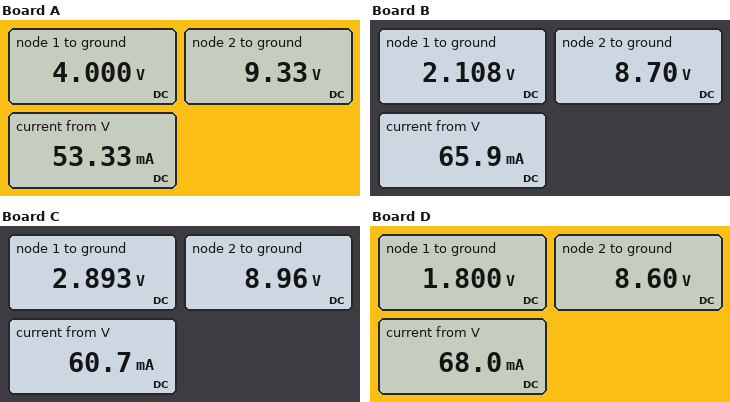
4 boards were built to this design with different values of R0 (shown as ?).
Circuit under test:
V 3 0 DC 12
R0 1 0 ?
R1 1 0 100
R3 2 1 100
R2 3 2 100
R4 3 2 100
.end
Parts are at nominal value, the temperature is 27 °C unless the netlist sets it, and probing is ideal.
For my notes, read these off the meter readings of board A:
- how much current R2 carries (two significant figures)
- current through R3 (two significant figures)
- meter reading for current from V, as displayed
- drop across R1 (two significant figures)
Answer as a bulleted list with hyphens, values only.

- 27 mA
- 53 mA
- 53.33 mA
- 4.0 V
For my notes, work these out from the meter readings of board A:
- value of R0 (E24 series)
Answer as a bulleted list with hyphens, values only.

- 300 Ω
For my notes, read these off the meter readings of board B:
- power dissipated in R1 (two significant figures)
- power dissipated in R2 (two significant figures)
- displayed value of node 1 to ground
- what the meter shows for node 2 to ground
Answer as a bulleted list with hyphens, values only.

- 44 mW
- 110 mW
- 2.108 V
- 8.70 V
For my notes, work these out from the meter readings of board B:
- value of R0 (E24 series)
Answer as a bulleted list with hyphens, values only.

- 47 Ω
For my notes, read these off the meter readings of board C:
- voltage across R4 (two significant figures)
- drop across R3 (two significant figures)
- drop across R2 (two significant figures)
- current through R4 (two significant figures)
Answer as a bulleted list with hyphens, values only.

- 3.0 V
- 6.1 V
- 3.0 V
- 30 mA
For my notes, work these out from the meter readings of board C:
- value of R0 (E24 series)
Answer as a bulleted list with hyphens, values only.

- 91 Ω
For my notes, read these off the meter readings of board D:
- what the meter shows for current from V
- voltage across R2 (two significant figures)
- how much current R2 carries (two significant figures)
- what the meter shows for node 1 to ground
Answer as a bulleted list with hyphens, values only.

- 68.0 mA
- 3.4 V
- 34 mA
- 1.800 V
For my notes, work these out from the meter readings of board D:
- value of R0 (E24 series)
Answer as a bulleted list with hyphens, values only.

- 36 Ω
